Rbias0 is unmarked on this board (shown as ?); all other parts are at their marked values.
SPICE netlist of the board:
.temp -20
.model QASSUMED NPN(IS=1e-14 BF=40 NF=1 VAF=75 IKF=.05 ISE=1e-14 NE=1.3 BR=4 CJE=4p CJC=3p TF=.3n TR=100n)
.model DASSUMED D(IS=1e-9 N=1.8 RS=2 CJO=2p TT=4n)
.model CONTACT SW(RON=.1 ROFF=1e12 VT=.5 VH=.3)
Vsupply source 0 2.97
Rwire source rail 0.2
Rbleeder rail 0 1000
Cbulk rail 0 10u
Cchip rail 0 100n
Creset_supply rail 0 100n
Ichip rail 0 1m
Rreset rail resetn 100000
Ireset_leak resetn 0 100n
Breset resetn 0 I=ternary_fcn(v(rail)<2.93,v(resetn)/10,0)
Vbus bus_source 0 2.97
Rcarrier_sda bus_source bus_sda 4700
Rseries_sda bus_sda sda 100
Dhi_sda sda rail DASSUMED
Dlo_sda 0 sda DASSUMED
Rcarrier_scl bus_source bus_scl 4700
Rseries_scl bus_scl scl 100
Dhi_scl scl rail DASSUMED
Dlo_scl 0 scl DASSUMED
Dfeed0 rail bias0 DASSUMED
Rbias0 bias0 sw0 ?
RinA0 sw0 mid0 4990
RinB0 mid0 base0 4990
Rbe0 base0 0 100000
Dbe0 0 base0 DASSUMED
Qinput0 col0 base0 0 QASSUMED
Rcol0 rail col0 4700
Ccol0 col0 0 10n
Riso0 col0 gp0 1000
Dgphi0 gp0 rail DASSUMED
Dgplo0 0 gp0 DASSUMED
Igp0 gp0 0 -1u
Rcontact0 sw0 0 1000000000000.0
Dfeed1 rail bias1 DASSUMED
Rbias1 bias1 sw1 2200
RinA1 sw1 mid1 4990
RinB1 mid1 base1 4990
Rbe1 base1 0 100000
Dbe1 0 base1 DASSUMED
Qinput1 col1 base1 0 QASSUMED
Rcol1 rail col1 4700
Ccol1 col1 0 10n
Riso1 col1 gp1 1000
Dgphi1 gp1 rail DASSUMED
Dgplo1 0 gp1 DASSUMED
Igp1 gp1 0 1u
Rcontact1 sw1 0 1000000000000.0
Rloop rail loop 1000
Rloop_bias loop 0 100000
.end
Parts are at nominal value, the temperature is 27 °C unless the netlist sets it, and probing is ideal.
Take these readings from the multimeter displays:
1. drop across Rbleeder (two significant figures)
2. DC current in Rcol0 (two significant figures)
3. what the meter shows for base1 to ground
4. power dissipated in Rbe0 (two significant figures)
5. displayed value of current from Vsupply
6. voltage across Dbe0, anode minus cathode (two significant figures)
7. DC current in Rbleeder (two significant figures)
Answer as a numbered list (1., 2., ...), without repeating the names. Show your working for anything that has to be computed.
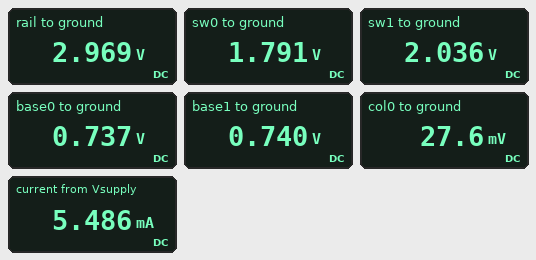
1. 2.969 V = 3.0 V
2. (2.969 V - 27.6 mV) / 4.7 kΩ = 630 µA
3. 0.740 V
4. (737 mV)^2 / 100 kΩ = 5.4 µW
5. 5.486 mA
6. 0 V - 737 mV = -740 mV
7. (2.969 V) / 1 kΩ = 3.0 mA
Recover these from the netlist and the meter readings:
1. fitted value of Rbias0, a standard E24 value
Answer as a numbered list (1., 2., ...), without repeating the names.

1. 5.1 kΩ
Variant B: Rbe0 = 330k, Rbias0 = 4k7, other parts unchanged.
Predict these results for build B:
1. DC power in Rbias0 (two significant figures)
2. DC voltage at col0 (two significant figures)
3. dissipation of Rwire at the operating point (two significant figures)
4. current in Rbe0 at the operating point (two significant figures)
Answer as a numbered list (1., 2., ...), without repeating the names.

1. 55 µW
2. 26 mV
3. 6.0 µW
4. 2.2 µA
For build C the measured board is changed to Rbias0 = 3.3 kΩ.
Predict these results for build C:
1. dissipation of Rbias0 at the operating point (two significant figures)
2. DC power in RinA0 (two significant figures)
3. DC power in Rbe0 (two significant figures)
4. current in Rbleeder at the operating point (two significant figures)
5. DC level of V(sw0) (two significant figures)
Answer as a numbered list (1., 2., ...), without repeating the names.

1. 47 µW
2. 71 µW
3. 5.5 µW
4. 3.0 mA
5. 1.9 V
